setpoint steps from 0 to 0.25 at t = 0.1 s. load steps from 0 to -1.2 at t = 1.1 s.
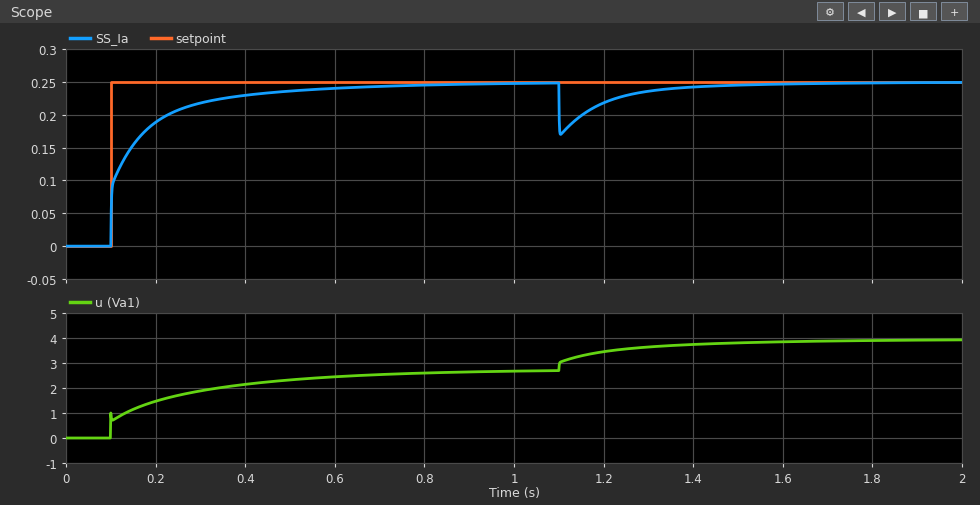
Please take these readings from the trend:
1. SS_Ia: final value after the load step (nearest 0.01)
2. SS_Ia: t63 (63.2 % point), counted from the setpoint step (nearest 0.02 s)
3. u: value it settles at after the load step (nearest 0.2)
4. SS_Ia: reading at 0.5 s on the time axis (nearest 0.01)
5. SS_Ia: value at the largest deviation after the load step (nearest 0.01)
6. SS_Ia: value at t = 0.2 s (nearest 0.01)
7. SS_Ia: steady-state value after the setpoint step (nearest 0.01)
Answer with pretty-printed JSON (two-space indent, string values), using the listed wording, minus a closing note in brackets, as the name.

{
  "SS_Ia: final value after the load step": "0.25",
  "SS_Ia: t63 (63.2 % point), counted from the setpoint step": "0.06 s",
  "u: value it settles at after the load step": "4.0",
  "SS_Ia: reading at 0.5 s on the time axis": "0.24",
  "SS_Ia: value at the largest deviation after the load step": "0.17",
  "SS_Ia: value at t = 0.2 s": "0.19",
  "SS_Ia: steady-state value after the setpoint step": "0.25"
}
